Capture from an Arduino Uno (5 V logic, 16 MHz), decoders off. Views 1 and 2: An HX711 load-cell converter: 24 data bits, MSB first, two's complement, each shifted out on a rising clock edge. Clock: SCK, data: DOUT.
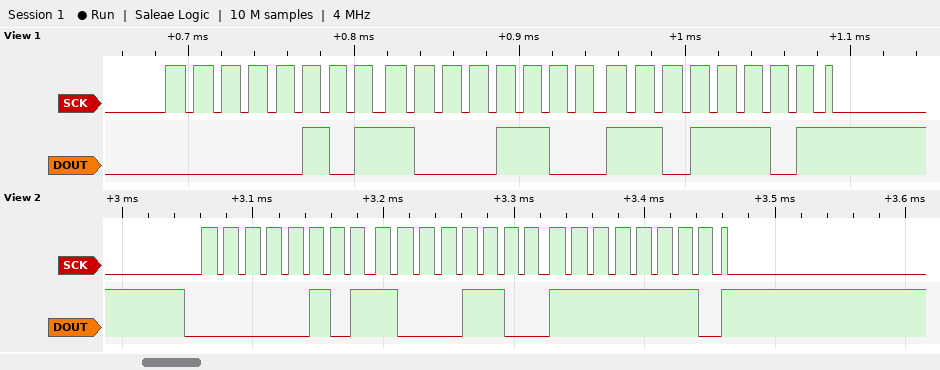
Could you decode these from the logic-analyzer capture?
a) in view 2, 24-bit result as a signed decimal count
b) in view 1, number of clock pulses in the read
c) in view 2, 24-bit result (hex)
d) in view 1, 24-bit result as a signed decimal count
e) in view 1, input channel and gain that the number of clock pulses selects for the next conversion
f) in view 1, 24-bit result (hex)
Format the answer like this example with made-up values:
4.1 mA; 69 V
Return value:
363774; 25; 0x058CFE; 363741; channel A, gain 128; 0x058CDD
